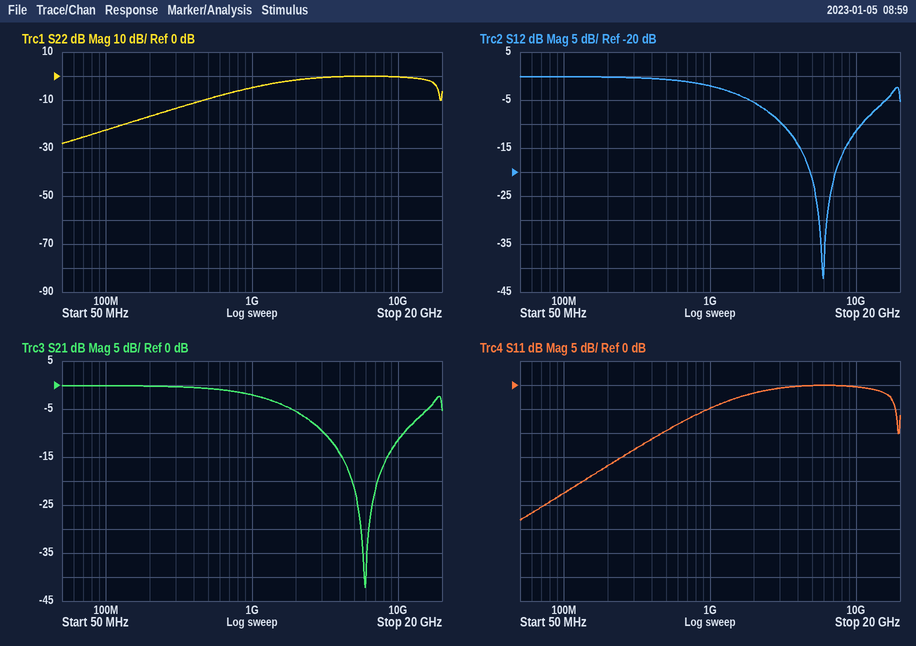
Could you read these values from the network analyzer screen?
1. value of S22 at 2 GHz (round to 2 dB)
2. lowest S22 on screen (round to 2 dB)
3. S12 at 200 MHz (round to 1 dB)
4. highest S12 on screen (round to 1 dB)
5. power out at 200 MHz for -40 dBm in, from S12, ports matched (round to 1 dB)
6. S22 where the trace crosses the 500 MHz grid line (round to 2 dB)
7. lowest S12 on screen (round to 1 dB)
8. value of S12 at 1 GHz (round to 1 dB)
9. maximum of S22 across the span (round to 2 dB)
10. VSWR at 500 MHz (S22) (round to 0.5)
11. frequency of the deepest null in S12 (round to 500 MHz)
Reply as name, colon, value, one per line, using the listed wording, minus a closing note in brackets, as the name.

value of S22 at 2 GHz: -2 dB
lowest S22 on screen: -28 dB
S12 at 200 MHz: 0 dB
highest S12 on screen: 0 dB
power out at 200 MHz for -40 dBm in, from S12, ports matched: -40 dBm
S22 where the trace crosses the 500 MHz grid line: -10 dB
lowest S12 on screen: -42 dB
value of S12 at 1 GHz: -2 dB
maximum of S22 across the span: 0 dB
VSWR at 500 MHz (S22): 2.0
frequency of the deepest null in S12: 6.0 GHz
